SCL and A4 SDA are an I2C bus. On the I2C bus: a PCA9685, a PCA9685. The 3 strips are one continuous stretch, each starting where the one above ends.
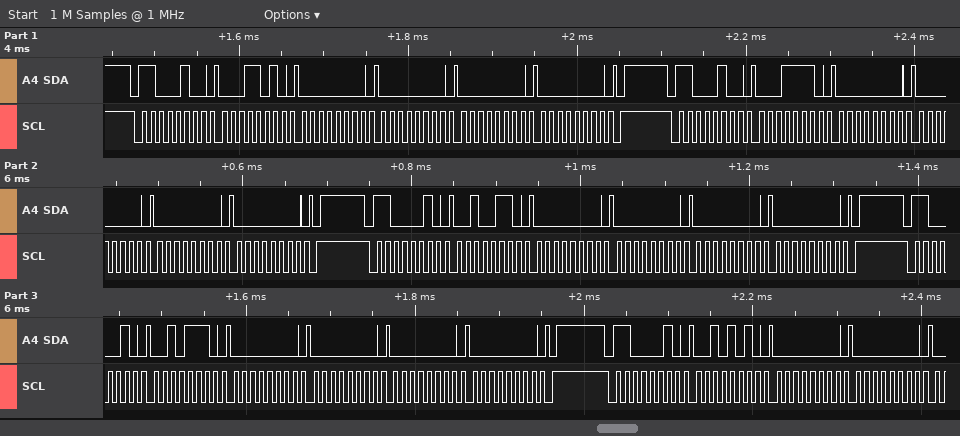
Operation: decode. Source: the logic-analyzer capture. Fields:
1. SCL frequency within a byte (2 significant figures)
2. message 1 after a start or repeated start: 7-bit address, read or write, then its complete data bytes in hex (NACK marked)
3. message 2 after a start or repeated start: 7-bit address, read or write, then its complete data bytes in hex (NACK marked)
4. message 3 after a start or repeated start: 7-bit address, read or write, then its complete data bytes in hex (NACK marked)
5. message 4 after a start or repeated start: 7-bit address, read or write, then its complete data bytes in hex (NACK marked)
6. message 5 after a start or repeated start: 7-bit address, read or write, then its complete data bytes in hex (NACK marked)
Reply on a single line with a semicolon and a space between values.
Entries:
100 kHz; 0x62 write: 1A 00 00 00 00; 0x62 write: 1E 00 00 00 00; 0x61 write: 26 00 00 00 00; 0x61 write: 2E 00 00 00 00; 0x61 write: 2A 00 00
